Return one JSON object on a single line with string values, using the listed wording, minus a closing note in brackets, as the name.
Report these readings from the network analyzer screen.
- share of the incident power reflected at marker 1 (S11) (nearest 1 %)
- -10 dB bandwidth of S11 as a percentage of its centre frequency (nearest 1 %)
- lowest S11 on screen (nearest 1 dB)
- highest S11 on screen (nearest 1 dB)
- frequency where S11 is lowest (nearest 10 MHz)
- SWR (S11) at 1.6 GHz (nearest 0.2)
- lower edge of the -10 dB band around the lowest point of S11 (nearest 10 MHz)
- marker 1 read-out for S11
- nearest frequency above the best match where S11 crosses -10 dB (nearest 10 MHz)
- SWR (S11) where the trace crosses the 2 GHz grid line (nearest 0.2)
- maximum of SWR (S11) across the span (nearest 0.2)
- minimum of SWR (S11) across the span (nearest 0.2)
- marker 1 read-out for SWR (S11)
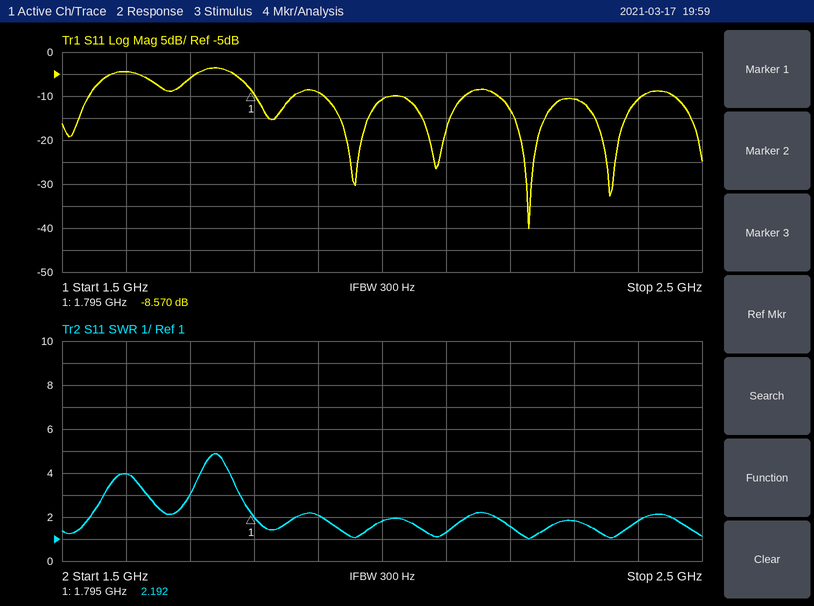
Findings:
{"share of the incident power reflected at marker 1 (S11)": "14 %", "-10 dB bandwidth of S11 as a percentage of its centre frequency": "10 %", "lowest S11 on screen": "-40 dB", "highest S11 on screen": "-4 dB", "frequency where S11 is lowest": "2.23 GHz", "SWR (S11) at 1.6 GHz": "4.0", "lower edge of the -10 dB band around the lowest point of S11": "2.18 GHz", "marker 1 read-out for S11": "-8.570 dB", "nearest frequency above the best match where S11 crosses -10 dB": "2.41 GHz", "SWR (S11) where the trace crosses the 2 GHz grid line": "1.8", "maximum of SWR (S11) across the span": "4.8", "minimum of SWR (S11) across the span": "1.0", "marker 1 read-out for SWR": "2.192"}
